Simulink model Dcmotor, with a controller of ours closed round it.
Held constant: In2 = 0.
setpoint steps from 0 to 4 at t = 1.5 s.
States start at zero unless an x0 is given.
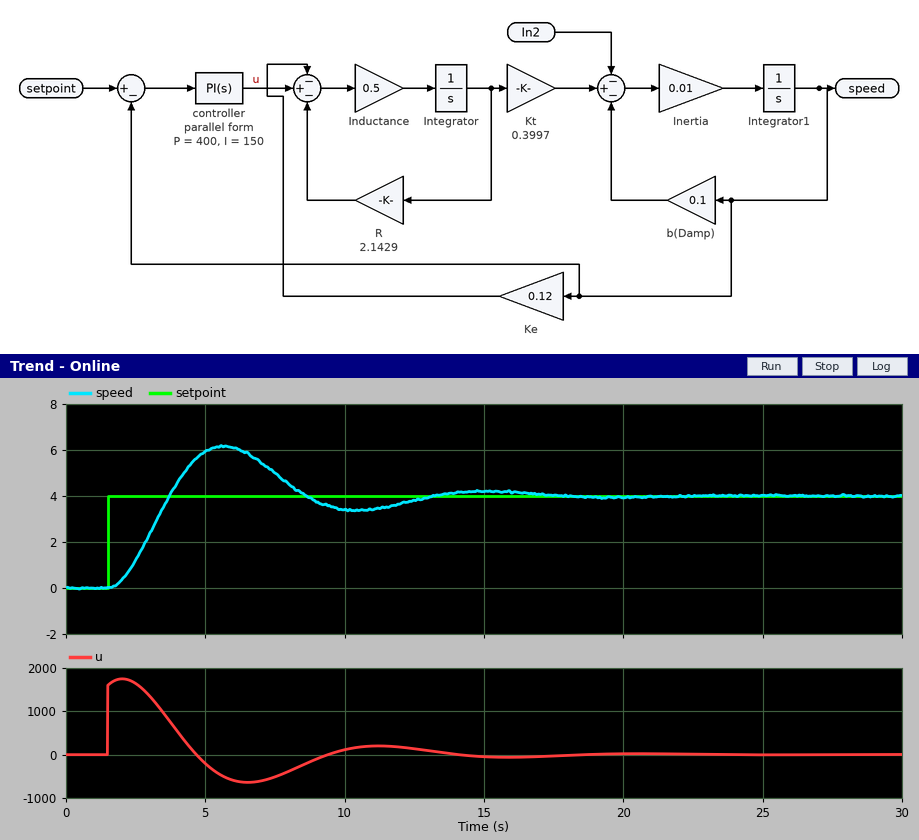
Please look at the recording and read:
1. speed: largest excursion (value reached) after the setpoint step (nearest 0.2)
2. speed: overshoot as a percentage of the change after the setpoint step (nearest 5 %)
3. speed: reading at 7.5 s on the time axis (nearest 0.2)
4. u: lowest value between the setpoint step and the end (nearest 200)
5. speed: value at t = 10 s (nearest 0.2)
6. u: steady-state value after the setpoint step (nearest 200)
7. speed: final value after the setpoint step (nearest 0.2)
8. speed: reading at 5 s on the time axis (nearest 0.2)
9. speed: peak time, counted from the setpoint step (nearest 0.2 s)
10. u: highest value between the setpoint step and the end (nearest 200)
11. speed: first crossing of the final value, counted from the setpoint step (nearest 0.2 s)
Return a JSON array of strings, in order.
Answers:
["6.2", "55 %", "5.0", "-600", "3.4", "0", "4.0", "6.0", "4.2 s", "1800", "2.2 s"]
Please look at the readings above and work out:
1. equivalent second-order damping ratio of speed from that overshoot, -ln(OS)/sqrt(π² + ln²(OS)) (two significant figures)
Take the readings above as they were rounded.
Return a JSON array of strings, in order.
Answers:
["0.19"]
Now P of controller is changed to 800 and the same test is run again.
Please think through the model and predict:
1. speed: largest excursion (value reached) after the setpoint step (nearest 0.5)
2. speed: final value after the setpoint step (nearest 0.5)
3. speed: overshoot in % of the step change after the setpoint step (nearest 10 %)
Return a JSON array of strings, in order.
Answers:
["5.5", "4.0", "40 %"]
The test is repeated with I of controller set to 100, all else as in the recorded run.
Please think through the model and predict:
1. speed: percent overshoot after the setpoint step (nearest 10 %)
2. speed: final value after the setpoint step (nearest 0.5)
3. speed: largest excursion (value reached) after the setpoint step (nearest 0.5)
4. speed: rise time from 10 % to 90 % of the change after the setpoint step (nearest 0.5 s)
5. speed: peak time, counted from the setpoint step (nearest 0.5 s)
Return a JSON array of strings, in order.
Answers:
["40 %", "4.0", "5.5", "1.5 s", "4.5 s"]
